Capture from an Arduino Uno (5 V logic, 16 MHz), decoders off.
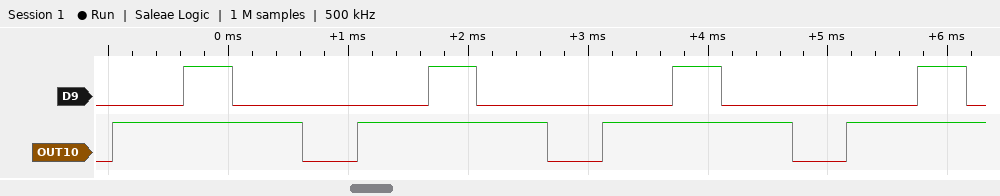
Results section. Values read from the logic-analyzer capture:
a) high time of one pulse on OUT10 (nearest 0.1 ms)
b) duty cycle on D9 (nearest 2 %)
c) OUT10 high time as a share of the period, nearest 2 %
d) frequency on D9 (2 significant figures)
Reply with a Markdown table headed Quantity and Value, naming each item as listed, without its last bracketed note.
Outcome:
| Quantity | Value |
|---|---|
| high time of one pulse on OUT10 | 1.6 ms |
| duty cycle on D9 | 20 % |
| OUT10 high time as a share of the period, nearest 2 % | 78 % |
| frequency on D9 | 490 Hz |
